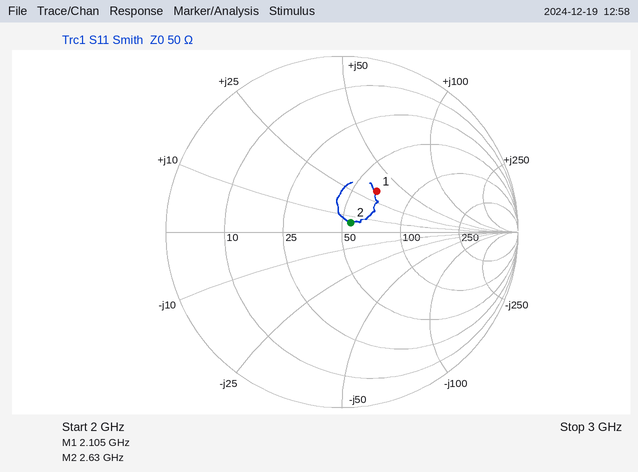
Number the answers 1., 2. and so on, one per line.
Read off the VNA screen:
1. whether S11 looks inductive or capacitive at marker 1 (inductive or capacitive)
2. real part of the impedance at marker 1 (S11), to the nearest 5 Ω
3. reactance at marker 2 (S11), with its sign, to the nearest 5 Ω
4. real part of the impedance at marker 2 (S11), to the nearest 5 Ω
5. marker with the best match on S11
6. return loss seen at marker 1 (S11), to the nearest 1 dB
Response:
1. inductive
2. 65 Ω
3. +5 Ω
4. 55 Ω
5. marker 2
6. 10 dB
